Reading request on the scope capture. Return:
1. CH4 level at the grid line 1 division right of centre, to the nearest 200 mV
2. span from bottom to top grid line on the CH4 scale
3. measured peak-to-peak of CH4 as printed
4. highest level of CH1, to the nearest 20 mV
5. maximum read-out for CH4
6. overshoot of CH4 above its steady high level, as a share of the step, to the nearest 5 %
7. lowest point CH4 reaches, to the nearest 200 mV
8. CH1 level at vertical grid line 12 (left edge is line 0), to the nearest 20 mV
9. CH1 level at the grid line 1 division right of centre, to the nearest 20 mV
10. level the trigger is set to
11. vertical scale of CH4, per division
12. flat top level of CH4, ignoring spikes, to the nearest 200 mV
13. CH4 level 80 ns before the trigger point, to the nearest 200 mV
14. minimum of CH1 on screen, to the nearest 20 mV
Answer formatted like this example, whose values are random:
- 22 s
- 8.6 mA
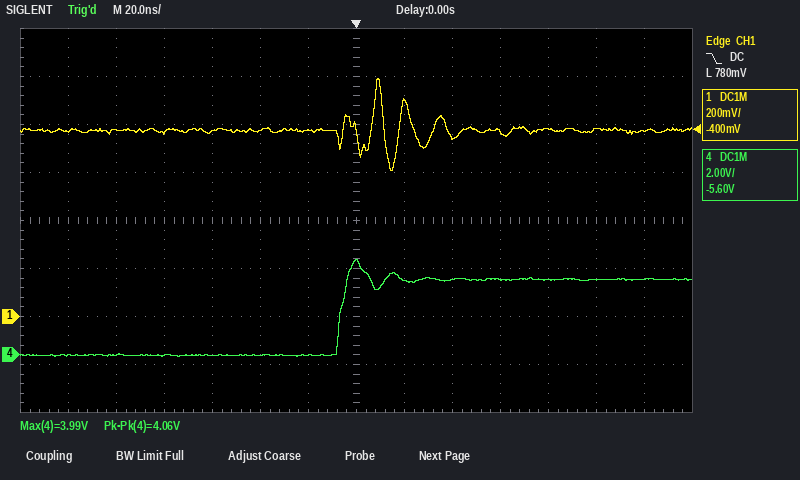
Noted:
- 3.2 V
- 16 V
- 4.06 V
- 1.00 V
- 3.99 V
- 25 %
- 0.0 V
- 780 mV
- 900 mV
- 780 mV
- 2 V
- 3.2 V
- 0.0 V
- 600 mV
